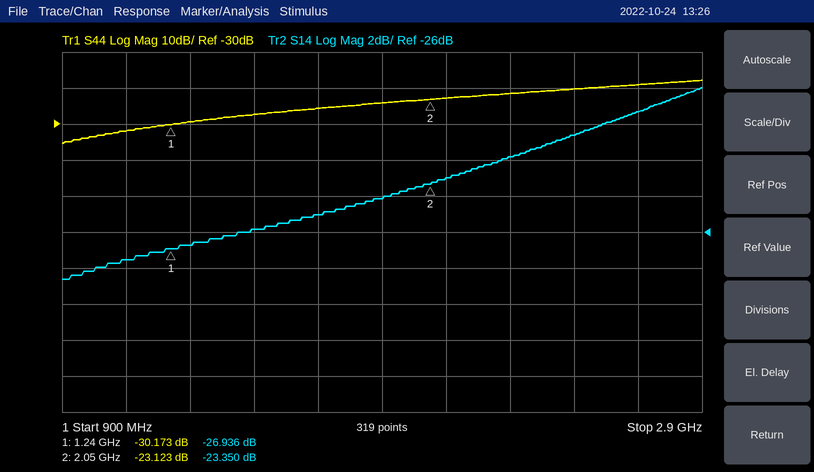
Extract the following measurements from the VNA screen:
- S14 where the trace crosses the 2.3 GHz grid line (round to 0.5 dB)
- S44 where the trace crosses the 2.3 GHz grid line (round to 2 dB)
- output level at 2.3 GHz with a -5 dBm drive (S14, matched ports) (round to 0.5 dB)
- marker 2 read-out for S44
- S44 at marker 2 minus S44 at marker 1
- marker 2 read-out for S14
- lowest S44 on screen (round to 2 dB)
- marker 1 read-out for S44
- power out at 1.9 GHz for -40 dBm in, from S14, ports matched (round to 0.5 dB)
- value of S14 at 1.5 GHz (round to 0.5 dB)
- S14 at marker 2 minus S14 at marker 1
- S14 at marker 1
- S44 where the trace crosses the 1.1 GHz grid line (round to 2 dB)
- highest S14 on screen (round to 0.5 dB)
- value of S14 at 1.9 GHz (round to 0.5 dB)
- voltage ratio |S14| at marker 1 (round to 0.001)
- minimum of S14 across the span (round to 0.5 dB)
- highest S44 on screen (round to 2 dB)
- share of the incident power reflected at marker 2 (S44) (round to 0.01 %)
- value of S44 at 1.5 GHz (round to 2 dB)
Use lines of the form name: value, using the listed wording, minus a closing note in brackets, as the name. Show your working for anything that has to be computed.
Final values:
S14 where the trace crosses the 2.3 GHz grid line: -22.0 dB
S44 where the trace crosses the 2.3 GHz grid line: -22 dB
output level at 2.3 GHz with a -5 dBm drive (S14, matched ports): -5 dBm + (-22.0 dB) = -27.0 dBm
marker 2 read-out for S44: -23.123 dB
S44 at marker 2 minus S44 at marker 1: -23.123 − (-30.173) = 7.050 dB
marker 2 read-out for S14: -23.350 dB
lowest S44 on screen: -36 dB
marker 1 read-out for S44: -30.173 dB
power out at 1.9 GHz for -40 dBm in, from S14, ports matched: -40 dBm + (-24.0 dB) = -64.0 dBm
value of S14 at 1.5 GHz: -26.0 dB
S14 at marker 2 minus S14 at marker 1: -23.35 − (-26.936) = 3.586 dB
S14 at marker 1: -26.936 dB
S44 where the trace crosses the 1.1 GHz grid line: -32 dB
highest S14 on screen: -18.0 dB
value of S14 at 1.9 GHz: -24.0 dB
voltage ratio |S14| at marker 1: 10^(-26.936/20) ≈ 0.045
minimum of S14 across the span: -28.5 dB
highest S44 on screen: -18 dB
share of the incident power reflected at marker 2 (S44): 10^(-23.123/10) ≈ 0.49 %
value of S44 at 1.5 GHz: -28 dB
